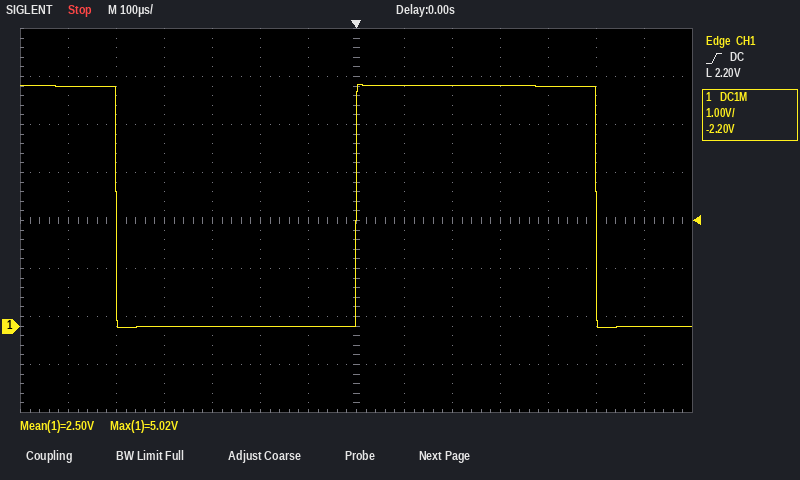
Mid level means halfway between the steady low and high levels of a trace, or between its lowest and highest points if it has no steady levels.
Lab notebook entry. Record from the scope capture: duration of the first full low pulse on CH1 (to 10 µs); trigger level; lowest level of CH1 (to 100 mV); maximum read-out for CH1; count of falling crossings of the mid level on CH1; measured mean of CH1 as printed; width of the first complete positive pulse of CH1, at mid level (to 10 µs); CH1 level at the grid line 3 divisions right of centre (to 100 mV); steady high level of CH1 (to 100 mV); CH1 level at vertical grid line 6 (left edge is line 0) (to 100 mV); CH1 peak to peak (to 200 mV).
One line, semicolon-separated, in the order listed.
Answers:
500 µs; 2.20 V; 0.0 V; 5.02 V; 2; 2.50 V; 500 µs; 5.0 V; 5.0 V; 0.0 V; 5.0 V
